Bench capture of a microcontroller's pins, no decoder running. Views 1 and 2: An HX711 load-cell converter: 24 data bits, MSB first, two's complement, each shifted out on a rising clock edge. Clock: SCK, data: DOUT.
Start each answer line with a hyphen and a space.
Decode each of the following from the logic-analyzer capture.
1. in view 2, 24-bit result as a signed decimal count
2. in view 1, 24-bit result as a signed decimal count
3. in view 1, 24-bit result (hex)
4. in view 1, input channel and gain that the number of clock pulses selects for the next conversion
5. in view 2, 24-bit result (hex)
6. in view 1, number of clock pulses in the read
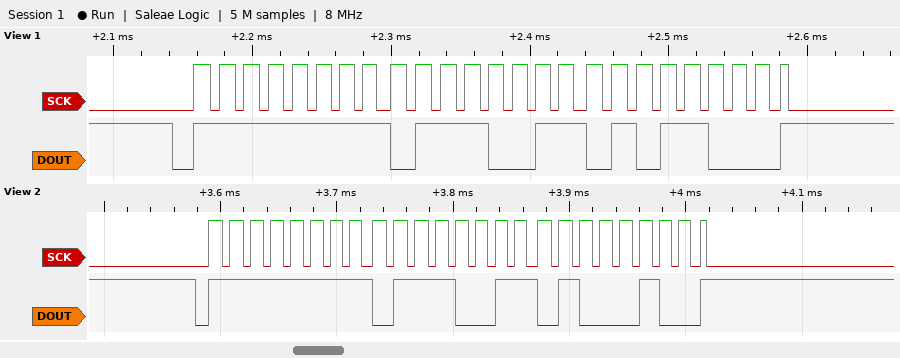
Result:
- -36028
- -36008
- 0xFF7358
- channel A, gain 128
- 0xFF7344
- 25
